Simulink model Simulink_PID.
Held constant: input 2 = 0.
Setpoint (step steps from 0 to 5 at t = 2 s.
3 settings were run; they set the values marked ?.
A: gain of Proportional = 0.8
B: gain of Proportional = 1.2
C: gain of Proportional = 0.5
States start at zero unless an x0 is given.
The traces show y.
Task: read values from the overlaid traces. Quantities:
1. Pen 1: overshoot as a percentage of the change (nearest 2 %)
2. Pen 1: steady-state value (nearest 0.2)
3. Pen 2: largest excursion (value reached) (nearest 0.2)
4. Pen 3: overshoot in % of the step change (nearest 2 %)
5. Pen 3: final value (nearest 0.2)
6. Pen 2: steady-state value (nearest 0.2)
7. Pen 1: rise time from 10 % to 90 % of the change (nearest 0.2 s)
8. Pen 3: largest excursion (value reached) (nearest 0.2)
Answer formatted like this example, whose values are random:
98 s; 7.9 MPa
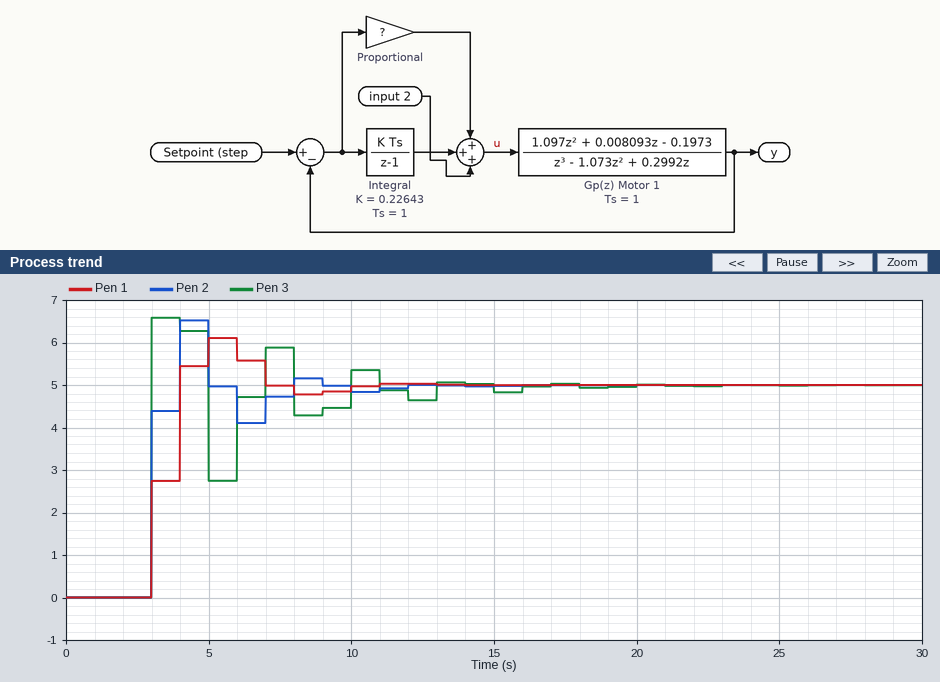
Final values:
22 %; 5.0; 6.6; 32 %; 5.0; 5.0; 1.0 s; 6.6
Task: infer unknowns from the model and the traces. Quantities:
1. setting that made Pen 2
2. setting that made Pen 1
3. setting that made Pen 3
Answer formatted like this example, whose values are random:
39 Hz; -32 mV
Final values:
A; C; B
